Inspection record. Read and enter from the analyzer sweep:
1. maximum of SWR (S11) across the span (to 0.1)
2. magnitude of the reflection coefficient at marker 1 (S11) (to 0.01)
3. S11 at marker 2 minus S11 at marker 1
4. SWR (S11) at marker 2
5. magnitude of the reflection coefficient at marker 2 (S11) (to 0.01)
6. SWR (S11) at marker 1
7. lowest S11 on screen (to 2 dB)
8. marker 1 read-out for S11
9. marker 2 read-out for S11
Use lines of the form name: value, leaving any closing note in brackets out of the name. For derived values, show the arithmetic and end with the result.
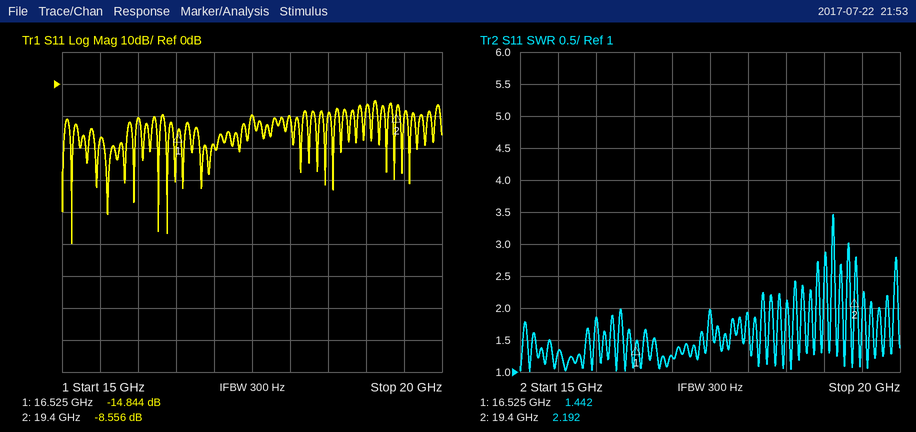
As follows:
maximum of SWR (S11) across the span: 3.5
magnitude of the reflection coefficient at marker 1 (S11): 10^(-14.844/20) ≈ 0.18
S11 at marker 2 minus S11 at marker 1: -8.556 − (-14.844) = 6.288 dB
SWR (S11) at marker 2: 2.192
magnitude of the reflection coefficient at marker 2 (S11): 10^(-8.556/20) ≈ 0.37
SWR (S11) at marker 1: 1.442
lowest S11 on screen: -50 dB
marker 1 read-out for S11: -14.844 dB
marker 2 read-out for S11: -8.556 dB
